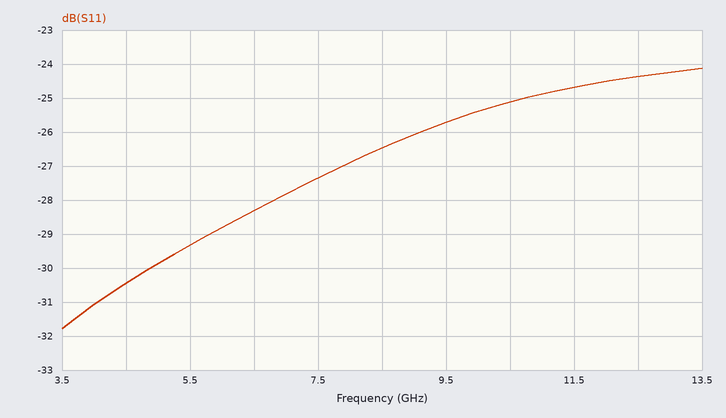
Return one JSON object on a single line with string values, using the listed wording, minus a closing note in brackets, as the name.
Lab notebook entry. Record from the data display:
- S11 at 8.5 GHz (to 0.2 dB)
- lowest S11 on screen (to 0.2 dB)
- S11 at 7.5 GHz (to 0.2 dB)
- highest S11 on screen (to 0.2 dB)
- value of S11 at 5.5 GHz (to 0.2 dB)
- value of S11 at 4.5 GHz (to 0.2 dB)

{"S11 at 8.5 GHz": "-26.4 dB", "lowest S11 on screen": "-31.8 dB", "S11 at 7.5 GHz": "-27.4 dB", "highest S11 on screen": "-24.2 dB", "value of S11 at 5.5 GHz": "-29.4 dB", "value of S11 at 4.5 GHz": "-30.4 dB"}
